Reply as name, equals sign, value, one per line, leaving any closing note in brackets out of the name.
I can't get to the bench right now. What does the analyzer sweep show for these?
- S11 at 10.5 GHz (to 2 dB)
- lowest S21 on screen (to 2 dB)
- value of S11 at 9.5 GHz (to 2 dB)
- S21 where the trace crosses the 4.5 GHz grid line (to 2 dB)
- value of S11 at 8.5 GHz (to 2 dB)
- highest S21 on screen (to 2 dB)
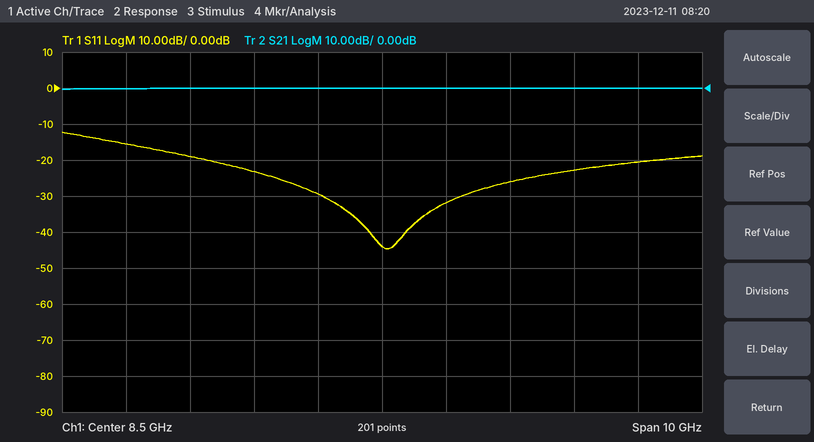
S11 at 10.5 GHz = -26 dB
lowest S21 on screen = 0 dB
value of S11 at 9.5 GHz = -32 dB
S21 where the trace crosses the 4.5 GHz grid line = 0 dB
value of S11 at 8.5 GHz = -44 dB
highest S21 on screen = 0 dB
